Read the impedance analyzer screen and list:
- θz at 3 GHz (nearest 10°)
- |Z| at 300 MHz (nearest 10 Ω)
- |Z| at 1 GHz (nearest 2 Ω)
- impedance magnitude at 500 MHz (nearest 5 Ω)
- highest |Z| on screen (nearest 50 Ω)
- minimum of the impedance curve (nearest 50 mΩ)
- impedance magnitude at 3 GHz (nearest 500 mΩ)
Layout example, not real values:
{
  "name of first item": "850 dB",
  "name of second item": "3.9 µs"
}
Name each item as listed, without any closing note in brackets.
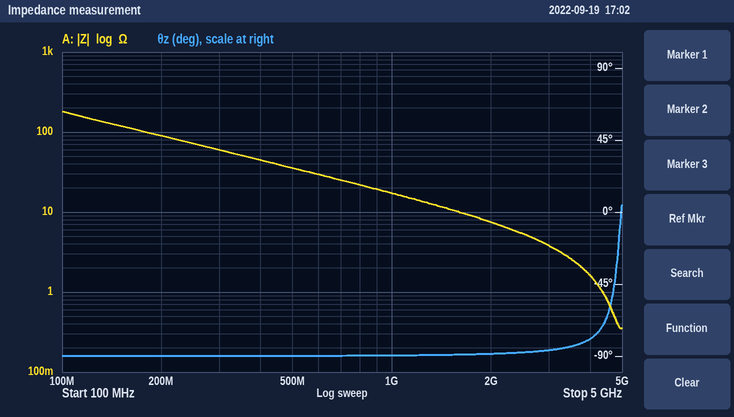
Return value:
{
  "θz at 3 GHz": "-90°",
  "|Z| at 300 MHz": "60 Ω",
  "|Z| at 1 GHz": "18 Ω",
  "impedance magnitude at 500 MHz": "35 Ω",
  "highest |Z| on screen": "200 Ω",
  "minimum of the impedance curve": "350 mΩ",
  "impedance magnitude at 3 GHz": "4.0 Ω"
}
